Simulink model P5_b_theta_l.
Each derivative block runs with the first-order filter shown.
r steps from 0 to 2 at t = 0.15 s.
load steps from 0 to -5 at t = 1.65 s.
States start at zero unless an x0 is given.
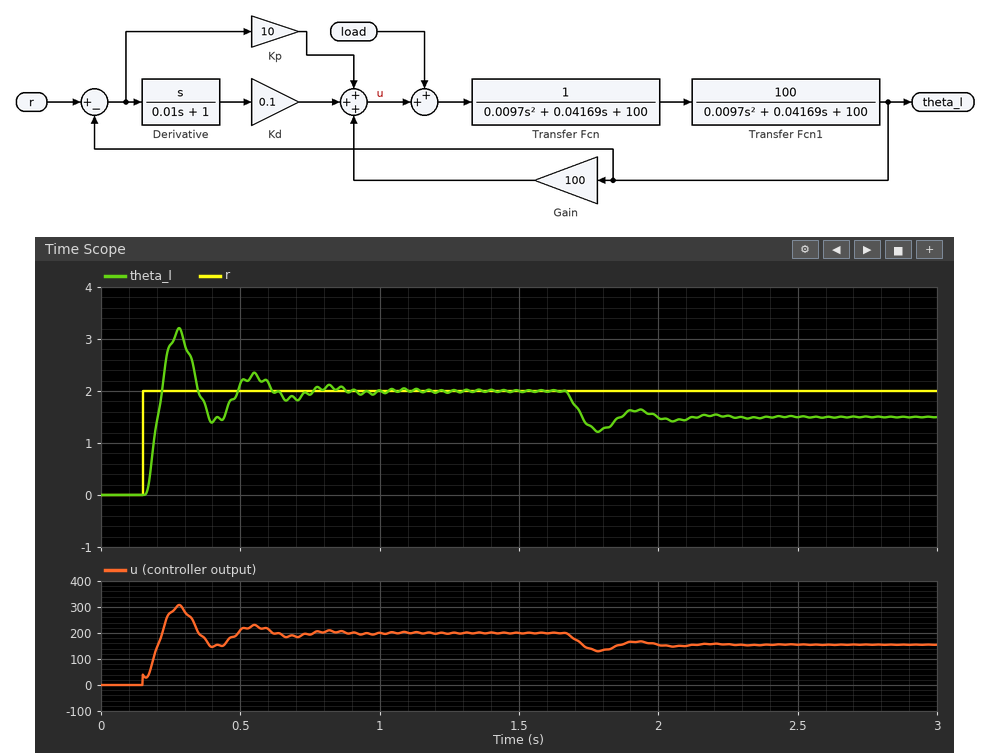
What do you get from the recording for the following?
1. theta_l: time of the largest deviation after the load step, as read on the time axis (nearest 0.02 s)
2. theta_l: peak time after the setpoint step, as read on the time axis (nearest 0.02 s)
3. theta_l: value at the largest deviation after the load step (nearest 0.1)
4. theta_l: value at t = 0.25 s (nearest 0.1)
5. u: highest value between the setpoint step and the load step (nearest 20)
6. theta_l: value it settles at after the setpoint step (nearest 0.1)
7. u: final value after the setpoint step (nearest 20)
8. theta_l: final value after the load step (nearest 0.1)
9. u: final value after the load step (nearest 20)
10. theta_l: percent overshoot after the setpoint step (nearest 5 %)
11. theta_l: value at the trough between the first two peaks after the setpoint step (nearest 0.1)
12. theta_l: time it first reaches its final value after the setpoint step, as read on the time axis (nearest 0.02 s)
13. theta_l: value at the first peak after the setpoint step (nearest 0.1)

1.78 s
0.28 s
1.2
2.9
300
2.0
200
1.5
160
60 %
1.4
0.22 s
3.2
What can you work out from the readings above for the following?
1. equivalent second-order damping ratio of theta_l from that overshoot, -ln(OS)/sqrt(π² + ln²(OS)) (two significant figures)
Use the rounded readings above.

0.16
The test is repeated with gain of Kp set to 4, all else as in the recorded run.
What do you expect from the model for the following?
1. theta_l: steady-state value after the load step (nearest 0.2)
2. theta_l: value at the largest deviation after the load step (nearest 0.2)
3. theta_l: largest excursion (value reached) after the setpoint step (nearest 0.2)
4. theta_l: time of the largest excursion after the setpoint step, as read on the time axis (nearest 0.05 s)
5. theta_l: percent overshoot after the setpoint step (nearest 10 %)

0.8
0.4
2.8
0.35 s
40 %
